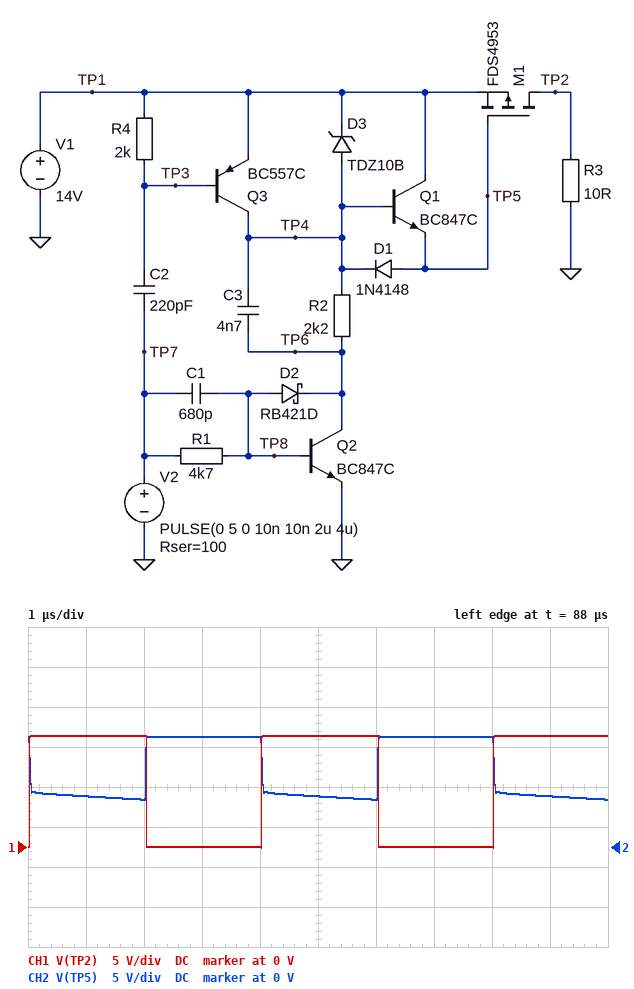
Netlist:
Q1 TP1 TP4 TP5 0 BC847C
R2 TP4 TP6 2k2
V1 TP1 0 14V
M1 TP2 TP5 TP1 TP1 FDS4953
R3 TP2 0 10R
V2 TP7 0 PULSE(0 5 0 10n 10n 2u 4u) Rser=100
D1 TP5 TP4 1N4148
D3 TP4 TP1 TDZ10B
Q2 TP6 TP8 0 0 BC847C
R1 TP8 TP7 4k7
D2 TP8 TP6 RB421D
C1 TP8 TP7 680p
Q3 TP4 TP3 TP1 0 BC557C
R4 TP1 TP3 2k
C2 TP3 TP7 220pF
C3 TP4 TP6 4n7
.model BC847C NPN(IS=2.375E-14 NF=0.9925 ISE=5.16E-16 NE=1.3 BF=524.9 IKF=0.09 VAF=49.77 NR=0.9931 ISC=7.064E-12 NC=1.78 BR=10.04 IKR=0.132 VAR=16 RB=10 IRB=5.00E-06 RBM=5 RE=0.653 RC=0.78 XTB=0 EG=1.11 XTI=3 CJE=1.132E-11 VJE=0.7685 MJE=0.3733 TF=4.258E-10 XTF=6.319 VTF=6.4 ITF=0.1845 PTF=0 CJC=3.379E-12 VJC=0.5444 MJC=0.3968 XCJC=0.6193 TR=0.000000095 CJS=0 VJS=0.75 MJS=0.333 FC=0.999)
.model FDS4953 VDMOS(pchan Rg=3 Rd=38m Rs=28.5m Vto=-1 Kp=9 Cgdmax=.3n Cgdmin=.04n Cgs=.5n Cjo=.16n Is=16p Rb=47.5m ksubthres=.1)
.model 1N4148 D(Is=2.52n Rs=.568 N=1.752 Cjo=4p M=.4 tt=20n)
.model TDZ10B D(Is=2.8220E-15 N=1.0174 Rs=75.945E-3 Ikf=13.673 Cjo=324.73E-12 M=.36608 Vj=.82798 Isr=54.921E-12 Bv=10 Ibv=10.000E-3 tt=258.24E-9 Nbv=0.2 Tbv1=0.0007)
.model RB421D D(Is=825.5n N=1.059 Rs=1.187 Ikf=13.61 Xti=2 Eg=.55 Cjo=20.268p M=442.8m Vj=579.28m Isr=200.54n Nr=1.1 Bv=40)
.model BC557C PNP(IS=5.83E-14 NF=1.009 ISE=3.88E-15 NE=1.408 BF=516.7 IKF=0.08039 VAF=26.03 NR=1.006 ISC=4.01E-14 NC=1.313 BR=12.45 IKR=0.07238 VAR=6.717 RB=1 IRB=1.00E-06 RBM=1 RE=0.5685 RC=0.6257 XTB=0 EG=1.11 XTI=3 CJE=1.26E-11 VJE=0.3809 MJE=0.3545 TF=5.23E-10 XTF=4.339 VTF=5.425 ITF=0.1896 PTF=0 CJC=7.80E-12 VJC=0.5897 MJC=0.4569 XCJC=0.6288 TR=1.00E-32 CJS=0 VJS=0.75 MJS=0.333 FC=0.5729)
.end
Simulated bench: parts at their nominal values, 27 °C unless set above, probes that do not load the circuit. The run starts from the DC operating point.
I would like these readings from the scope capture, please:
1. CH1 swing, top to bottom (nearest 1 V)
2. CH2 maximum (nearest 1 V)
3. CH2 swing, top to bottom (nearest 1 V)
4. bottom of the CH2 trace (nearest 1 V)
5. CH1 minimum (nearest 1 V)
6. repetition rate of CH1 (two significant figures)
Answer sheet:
14 V
14 V
8 V
6 V
0 V
250 kHz
